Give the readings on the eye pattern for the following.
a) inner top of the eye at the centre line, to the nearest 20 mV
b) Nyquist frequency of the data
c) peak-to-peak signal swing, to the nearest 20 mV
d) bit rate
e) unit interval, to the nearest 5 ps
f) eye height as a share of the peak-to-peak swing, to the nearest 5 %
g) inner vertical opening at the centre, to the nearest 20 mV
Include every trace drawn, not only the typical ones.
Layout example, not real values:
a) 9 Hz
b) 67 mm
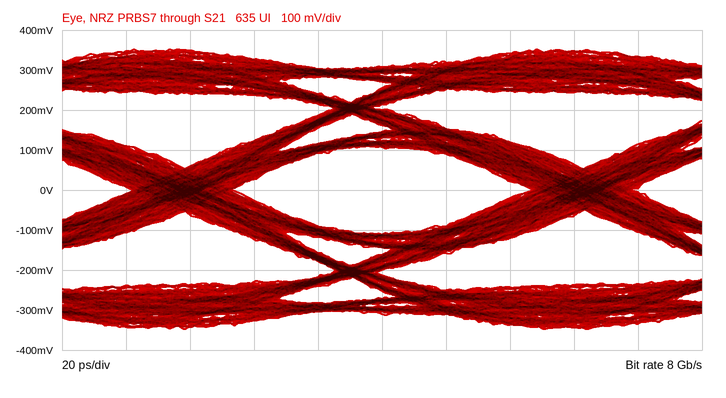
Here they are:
a) 100 mV
b) 4 GHz
c) 700 mV
d) 8 Gb/s
e) 125 ps
f) 30 %
g) 220 mV
